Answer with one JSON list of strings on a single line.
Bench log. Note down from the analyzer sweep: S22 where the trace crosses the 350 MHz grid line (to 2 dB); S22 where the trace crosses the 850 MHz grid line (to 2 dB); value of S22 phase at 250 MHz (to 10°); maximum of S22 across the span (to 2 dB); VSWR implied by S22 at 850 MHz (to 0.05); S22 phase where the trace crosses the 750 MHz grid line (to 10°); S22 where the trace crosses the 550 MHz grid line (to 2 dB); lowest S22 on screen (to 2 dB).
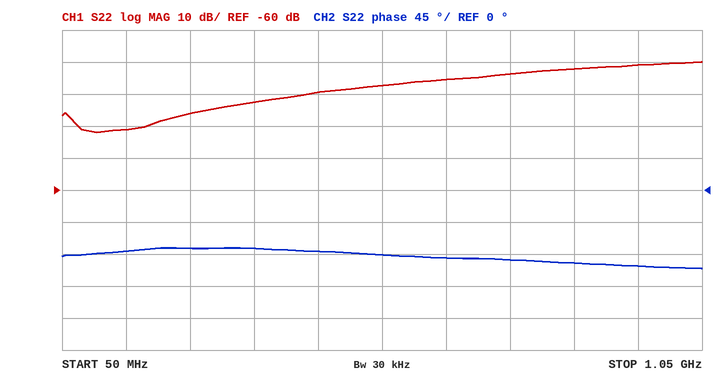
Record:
["-32 dB", "-22 dB", "-80°", "-20 dB", "1.15", "-100°", "-28 dB", "-42 dB"]
